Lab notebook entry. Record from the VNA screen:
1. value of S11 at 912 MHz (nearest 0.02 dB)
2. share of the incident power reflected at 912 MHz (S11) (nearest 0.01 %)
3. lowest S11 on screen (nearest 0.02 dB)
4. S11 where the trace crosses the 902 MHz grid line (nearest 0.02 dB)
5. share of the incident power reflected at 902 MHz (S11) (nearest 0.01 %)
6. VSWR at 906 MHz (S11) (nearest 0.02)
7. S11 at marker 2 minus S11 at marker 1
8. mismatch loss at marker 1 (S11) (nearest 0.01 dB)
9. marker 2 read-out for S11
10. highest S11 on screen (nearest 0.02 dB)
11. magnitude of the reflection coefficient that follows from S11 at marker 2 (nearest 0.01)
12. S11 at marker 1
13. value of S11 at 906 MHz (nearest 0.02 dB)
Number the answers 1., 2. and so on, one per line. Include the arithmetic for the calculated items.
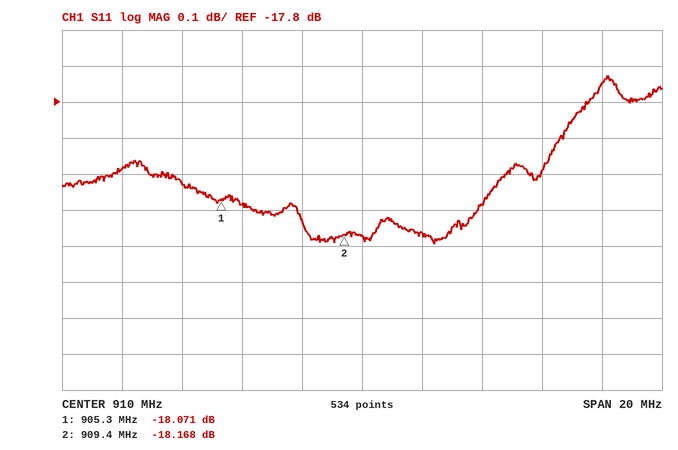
1. -18.16 dB
2. 10^(-18.16/10) ≈ 1.53 %
3. -18.20 dB
4. -17.98 dB
5. 10^(-17.98/10) ≈ 1.59 %
6. |Γ| = 10^(-18.08/20) = 0.1247; VSWR = (1 + 0.1247)/(1 − 0.1247) ≈ 1.29, so 1.28 to the nearest 0.02
7. -18.168 − (-18.071) = -0.097 dB
8. −10 log10(1 − 10^(-18.071/10)) ≈ 0.07 dB
9. -18.168 dB
10. -17.72 dB
11. 10^(-18.168/20) ≈ 0.12
12. -18.071 dB
13. -18.08 dB
